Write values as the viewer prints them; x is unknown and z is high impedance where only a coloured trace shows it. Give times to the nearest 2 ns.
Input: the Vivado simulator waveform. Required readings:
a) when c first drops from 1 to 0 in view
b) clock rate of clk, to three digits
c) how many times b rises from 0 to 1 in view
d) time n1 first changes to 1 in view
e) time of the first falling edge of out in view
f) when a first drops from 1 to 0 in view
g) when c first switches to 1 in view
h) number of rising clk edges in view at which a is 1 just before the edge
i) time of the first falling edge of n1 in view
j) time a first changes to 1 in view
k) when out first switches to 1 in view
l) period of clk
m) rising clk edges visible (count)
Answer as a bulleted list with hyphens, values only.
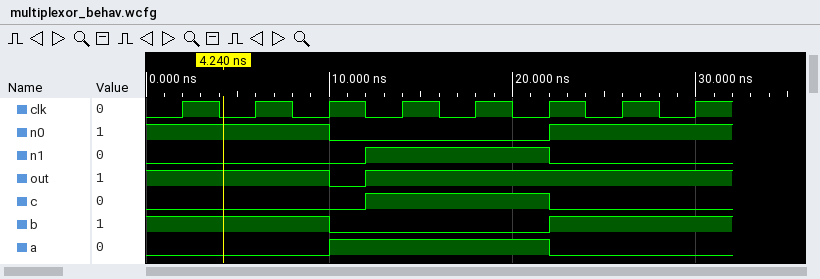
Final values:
- 22 ns
- 250 MHz
- 1
- 12 ns
- 10 ns
- 22 ns
- 12 ns
- 3
- 22 ns
- 10 ns
- 12 ns
- 4 ns
- 8
